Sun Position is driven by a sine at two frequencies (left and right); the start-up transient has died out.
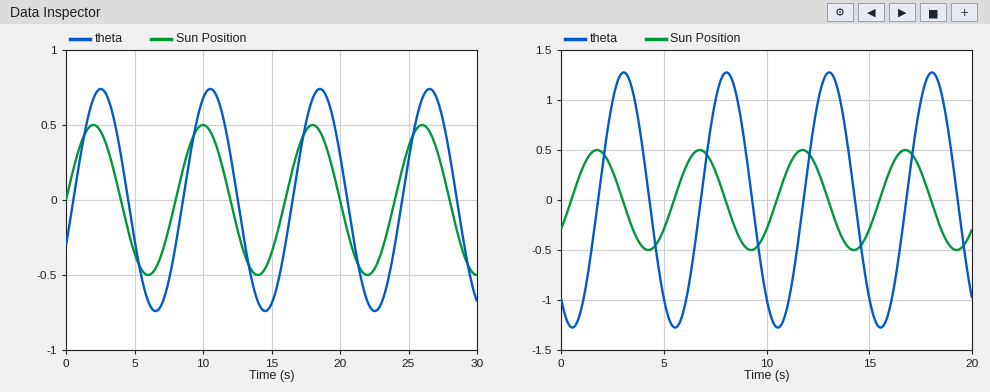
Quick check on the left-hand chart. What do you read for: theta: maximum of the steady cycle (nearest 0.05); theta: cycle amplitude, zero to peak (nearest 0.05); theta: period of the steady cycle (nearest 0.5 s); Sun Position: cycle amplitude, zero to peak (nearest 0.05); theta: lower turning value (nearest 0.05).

0.75
0.75
8.0 s
0.50
-0.75
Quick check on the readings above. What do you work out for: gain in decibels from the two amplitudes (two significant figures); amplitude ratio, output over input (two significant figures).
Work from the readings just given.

3.5 dB
1.5
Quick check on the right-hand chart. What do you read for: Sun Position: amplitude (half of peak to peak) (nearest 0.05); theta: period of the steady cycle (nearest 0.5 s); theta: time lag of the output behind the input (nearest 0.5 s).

0.50
5.0 s
1.5 s
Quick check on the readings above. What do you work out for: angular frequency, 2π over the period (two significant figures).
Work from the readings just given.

1.3 rad/s
